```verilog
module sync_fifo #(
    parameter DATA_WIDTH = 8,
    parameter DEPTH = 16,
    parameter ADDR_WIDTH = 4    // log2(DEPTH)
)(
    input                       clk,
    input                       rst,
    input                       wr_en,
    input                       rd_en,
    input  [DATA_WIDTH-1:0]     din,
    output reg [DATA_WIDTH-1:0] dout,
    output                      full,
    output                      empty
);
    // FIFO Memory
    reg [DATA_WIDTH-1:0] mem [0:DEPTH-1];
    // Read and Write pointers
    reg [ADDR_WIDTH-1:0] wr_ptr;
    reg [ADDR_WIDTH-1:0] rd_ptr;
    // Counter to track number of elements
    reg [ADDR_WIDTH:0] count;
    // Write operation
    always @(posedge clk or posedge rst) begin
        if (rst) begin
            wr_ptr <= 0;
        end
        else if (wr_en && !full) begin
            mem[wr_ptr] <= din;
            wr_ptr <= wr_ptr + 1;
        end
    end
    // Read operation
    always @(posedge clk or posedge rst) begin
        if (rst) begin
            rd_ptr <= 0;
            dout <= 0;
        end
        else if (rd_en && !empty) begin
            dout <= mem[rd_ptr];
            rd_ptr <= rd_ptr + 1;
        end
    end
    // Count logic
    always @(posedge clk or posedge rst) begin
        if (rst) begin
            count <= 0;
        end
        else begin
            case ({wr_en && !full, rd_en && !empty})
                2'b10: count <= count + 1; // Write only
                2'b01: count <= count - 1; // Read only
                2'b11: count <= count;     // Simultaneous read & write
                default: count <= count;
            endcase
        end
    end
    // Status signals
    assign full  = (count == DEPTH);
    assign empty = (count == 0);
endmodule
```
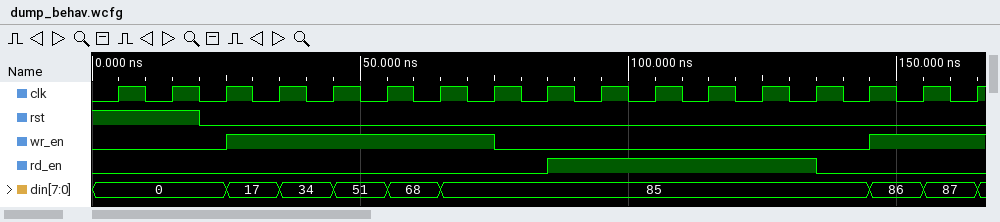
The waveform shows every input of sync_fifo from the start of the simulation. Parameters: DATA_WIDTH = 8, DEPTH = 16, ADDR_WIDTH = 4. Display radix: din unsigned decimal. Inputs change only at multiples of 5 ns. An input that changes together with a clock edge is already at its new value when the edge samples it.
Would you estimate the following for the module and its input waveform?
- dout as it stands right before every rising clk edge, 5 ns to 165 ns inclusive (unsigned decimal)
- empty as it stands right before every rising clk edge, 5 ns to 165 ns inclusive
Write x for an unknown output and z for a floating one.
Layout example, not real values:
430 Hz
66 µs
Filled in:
0, 0, 0, 0, 0, 0, 0, 0, 0, 17, 34, 51, 68, 85, 85, 85, 85
1 1 1 0 0 0 0 0 0 0 0 0 0 1 1 0 0
